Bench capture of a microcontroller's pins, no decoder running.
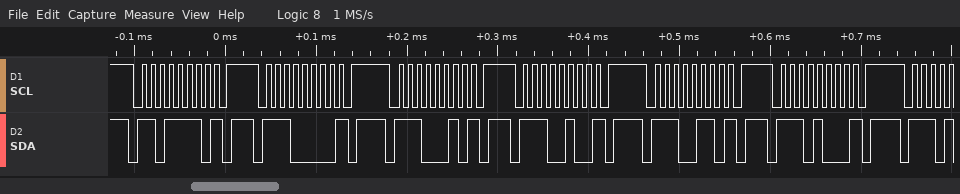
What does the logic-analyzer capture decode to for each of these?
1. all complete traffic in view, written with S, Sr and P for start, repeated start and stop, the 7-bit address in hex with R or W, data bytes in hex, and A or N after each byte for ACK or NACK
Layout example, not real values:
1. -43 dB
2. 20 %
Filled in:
1. S 6FW N P S 70W N P S 71W N P S 72W N P S 73W N P S 74W N P
